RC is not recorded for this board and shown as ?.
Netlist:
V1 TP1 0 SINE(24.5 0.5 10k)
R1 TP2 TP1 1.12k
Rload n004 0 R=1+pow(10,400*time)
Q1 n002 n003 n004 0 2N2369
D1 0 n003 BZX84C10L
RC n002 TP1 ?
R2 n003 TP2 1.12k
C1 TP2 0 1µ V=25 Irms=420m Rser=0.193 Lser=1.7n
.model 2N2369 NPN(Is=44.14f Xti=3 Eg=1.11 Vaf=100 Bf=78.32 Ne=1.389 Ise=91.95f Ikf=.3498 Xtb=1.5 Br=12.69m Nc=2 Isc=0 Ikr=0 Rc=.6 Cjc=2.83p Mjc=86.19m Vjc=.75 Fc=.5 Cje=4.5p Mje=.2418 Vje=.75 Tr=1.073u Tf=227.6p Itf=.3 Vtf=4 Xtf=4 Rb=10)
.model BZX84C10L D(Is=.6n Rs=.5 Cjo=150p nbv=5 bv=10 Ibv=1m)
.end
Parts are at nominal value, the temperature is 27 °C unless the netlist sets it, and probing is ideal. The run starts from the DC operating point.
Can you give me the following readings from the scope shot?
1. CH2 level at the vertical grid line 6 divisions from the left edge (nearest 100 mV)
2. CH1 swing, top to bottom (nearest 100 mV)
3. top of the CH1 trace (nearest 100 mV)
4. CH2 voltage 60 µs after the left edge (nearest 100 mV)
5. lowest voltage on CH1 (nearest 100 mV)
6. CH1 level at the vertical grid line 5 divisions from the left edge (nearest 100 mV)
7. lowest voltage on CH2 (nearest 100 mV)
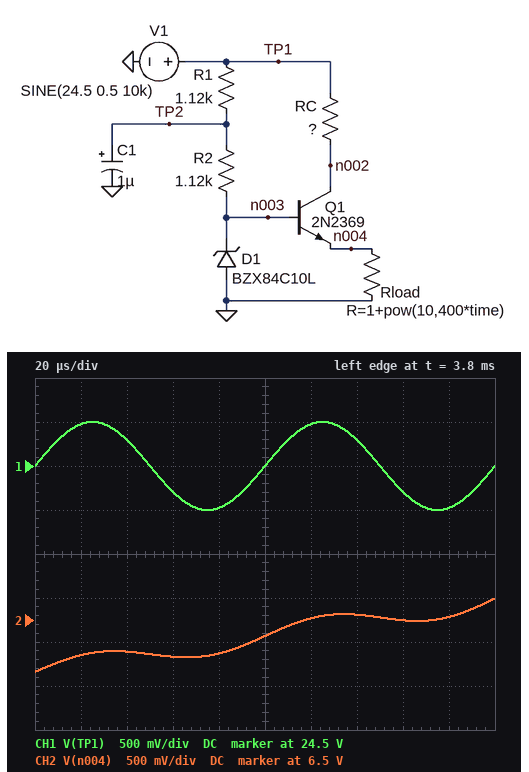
6.5 V
1.0 V
25.0 V
6.1 V
24.0 V
24.5 V
5.9 V
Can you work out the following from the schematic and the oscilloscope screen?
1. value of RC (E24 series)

110 Ω
